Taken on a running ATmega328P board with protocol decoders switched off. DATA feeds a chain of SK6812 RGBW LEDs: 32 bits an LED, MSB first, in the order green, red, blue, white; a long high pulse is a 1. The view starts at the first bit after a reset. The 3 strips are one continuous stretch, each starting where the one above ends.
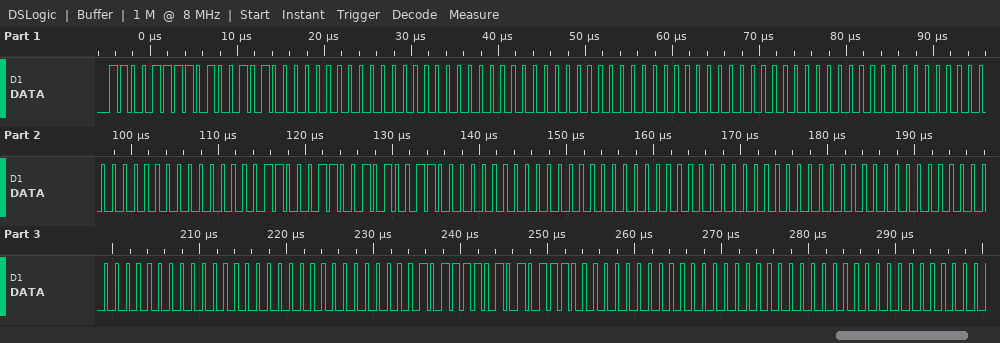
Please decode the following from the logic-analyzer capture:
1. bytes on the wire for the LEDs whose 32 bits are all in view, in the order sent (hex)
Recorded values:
CF 4A 00 00 00 00 00 00 00 00 00 00 C6 53 00 00 00 00 00 00 00 00 00 00 BD 5C 00 00
